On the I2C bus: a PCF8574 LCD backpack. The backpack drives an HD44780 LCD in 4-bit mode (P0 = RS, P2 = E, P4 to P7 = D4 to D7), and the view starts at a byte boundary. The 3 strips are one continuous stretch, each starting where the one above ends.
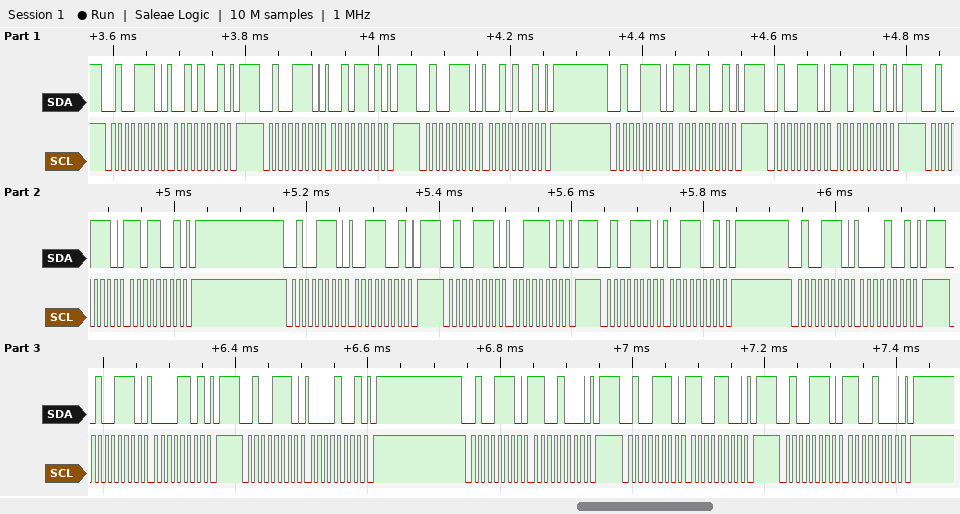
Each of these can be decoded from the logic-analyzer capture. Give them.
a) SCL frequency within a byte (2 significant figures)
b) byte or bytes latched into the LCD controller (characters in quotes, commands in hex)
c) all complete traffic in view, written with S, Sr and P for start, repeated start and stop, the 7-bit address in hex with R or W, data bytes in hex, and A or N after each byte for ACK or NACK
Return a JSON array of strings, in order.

["100 kHz", "'-' '0'", "S 27W A 29 A P S 27W A 2D A P S 27W A 29 A P S 27W A D9 A P S 27W A DD A P S 27W A D9 A P S 27W A 39 A P S 27W A 3D A P S 27W A 39 A P S 27W A 09 A P S 27W A 0D A P S 27W A 09 A P S 27W A C8 A P S 27W A CC A P S 27W A C8 A P"]
